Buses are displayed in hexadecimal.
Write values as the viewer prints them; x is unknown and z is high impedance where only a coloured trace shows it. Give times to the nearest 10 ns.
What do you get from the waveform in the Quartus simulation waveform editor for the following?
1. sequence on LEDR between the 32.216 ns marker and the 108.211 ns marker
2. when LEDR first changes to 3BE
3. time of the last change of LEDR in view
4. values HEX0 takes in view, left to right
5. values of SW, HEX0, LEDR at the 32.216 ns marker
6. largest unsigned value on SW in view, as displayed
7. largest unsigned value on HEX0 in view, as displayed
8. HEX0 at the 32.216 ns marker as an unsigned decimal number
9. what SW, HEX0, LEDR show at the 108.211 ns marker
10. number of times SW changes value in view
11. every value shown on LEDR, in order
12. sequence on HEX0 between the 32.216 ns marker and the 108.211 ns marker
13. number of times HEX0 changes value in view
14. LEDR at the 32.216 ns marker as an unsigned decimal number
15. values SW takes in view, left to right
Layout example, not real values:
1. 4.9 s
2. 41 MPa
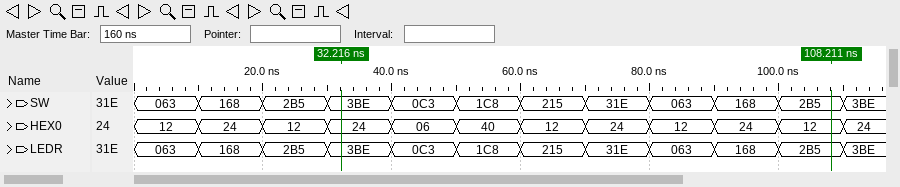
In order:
1. 3BE, 0C3, 1C8, 215, 31E, 063, 168, 2B5
2. 30 ns
3. 110 ns
4. 12, 24, 12, 24, 06, 40, 12, 24, 12, 24, 12, 24
5. SW=3BE, HEX0=24, LEDR=3BE
6. 3BE
7. 40
8. 36
9. SW=2B5, HEX0=12, LEDR=2B5
10. 11
11. 063, 168, 2B5, 3BE, 0C3, 1C8, 215, 31E, 063, 168, 2B5, 3BE
12. 24, 06, 40, 12, 24, 12, 24, 12
13. 11
14. 958
15. 063, 168, 2B5, 3BE, 0C3, 1C8, 215, 31E, 063, 168, 2B5, 3BE
